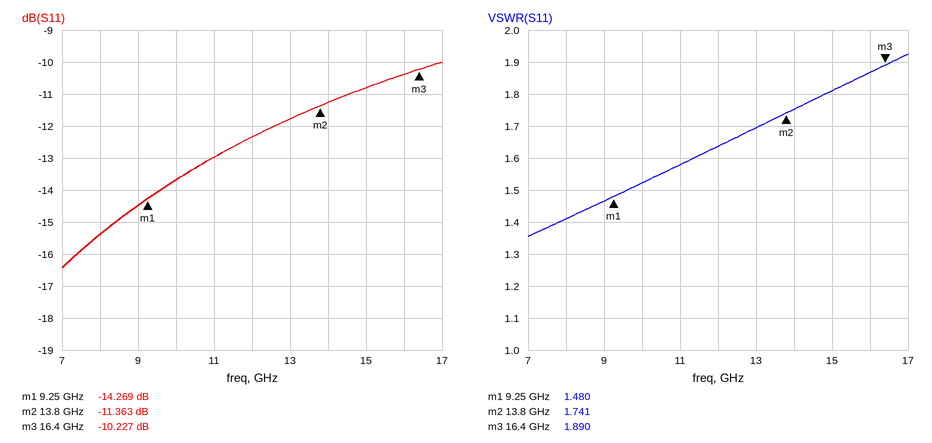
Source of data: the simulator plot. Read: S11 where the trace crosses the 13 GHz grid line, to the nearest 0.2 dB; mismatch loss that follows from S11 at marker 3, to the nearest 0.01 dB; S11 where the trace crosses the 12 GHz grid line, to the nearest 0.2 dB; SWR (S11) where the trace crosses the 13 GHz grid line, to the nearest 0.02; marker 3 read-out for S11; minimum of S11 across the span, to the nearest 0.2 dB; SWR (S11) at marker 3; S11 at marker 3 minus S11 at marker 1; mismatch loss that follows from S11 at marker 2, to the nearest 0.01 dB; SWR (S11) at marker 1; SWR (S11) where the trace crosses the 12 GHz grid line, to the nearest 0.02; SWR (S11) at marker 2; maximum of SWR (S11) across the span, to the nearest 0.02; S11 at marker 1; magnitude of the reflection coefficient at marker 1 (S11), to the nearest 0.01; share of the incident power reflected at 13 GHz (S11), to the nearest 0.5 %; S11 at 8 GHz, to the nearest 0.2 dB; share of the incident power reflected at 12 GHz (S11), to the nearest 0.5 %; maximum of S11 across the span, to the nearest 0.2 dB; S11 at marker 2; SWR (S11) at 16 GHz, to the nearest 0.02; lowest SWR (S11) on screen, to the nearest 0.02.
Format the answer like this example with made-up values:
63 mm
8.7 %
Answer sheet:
-11.8 dB
0.43 dB
-12.4 dB
1.70
-10.227 dB
-16.4 dB
1.890
4.042 dB
0.33 dB
1.480
1.64
1.741
1.92
-14.269 dB
0.19
6.5 %
-15.4 dB
6.0 %
-10.0 dB
-11.363 dB
1.86
1.36
